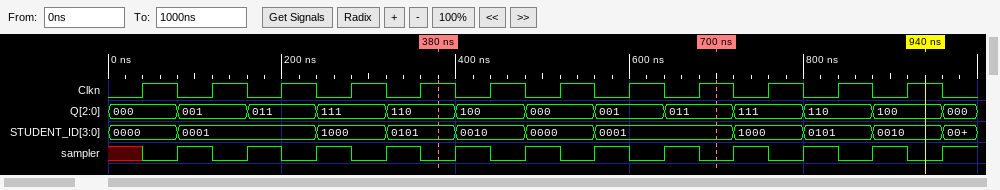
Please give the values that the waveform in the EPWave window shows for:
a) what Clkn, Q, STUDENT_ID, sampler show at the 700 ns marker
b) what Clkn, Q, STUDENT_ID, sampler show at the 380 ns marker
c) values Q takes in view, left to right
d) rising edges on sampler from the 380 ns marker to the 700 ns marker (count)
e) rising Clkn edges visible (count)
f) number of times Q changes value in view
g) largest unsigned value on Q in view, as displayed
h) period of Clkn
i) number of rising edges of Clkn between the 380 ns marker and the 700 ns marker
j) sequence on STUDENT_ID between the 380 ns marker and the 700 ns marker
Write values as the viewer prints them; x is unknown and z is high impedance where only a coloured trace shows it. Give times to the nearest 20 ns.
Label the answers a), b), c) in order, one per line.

a) Clkn=1, Q=011, STUDENT_ID=0001, sampler=0
b) Clkn=1, Q=110, STUDENT_ID=0101, sampler=0
c) 000, 001, 011, 111, 110, 100, 000, 001, 011, 111, 110, 100, 000
d) 4
e) 12
f) 12
g) 111
h) 80 ns
i) 4
j) 0101, 0010, 0000, 0001
